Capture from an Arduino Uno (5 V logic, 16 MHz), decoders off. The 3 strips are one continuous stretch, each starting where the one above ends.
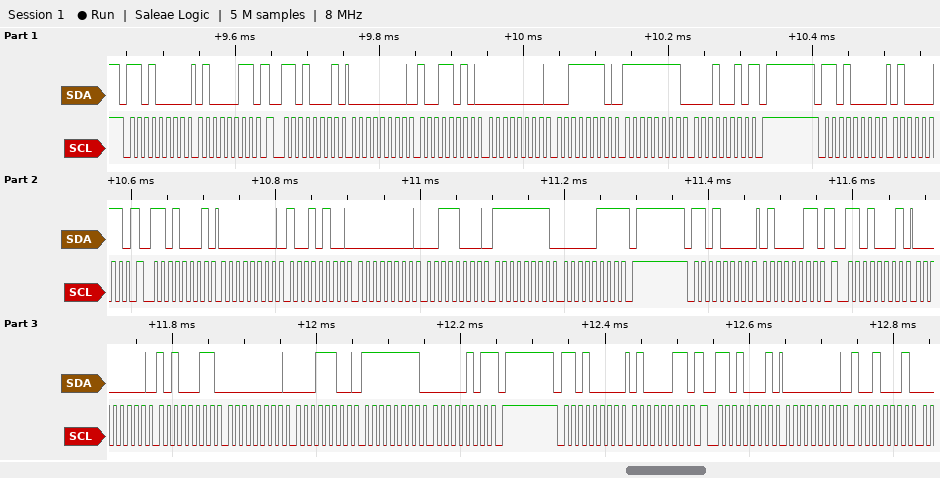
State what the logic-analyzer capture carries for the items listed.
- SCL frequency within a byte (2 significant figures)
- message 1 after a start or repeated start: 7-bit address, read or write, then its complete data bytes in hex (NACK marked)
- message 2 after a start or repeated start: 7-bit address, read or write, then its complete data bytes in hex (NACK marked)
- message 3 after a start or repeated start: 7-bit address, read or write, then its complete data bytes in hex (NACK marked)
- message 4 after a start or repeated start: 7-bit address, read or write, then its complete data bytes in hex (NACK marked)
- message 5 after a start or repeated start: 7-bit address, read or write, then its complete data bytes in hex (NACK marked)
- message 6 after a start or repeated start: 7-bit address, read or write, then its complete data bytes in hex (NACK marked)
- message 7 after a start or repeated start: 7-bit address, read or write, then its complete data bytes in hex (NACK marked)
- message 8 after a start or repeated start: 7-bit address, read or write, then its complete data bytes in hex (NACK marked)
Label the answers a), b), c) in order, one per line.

a) 100 kHz
b) 0x68 write: 43
c) 0x68 read: 00 9A 00 3E FF 12 NACK
d) 0x68 write: 43
e) 0x68 read: 00 94 00 38 FF 07 NACK
f) 0x68 write: 43
g) 0x68 read: 00 A3 00 1C FF 05 NACK
h) 0x68 write: 43
i) 0x68 read: 00 91
